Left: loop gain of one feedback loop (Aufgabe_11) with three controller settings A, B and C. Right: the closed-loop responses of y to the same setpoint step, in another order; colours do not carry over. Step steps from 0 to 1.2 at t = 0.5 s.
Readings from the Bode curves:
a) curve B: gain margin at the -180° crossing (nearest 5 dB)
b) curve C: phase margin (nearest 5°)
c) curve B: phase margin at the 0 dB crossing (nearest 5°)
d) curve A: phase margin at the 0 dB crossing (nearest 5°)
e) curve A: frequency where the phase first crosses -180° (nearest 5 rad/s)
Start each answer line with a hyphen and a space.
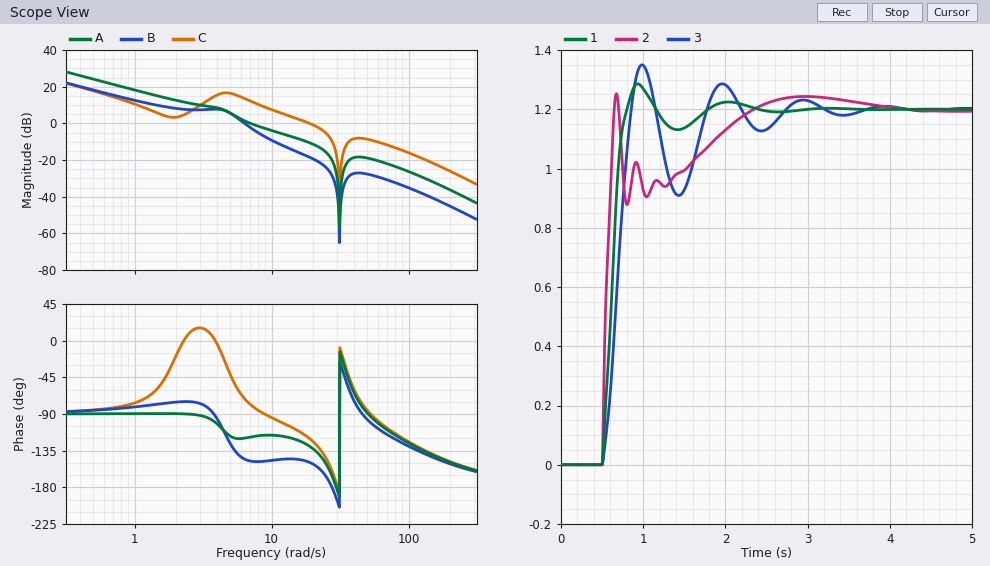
- 30 dB
- 60°
- 35°
- 60°
- 30 rad/s
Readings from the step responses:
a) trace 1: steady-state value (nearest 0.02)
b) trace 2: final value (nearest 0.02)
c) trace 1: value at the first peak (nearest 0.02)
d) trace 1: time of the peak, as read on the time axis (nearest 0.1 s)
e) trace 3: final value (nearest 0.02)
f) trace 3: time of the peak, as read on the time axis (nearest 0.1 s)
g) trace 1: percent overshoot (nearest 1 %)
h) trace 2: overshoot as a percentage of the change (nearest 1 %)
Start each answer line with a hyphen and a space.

- 1.20
- 1.20
- 1.28
- 0.9 s
- 1.20
- 1.0 s
- 7 %
- 4 %
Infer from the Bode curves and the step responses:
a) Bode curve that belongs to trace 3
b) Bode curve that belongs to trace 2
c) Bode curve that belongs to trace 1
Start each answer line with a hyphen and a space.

- B
- C
- A
